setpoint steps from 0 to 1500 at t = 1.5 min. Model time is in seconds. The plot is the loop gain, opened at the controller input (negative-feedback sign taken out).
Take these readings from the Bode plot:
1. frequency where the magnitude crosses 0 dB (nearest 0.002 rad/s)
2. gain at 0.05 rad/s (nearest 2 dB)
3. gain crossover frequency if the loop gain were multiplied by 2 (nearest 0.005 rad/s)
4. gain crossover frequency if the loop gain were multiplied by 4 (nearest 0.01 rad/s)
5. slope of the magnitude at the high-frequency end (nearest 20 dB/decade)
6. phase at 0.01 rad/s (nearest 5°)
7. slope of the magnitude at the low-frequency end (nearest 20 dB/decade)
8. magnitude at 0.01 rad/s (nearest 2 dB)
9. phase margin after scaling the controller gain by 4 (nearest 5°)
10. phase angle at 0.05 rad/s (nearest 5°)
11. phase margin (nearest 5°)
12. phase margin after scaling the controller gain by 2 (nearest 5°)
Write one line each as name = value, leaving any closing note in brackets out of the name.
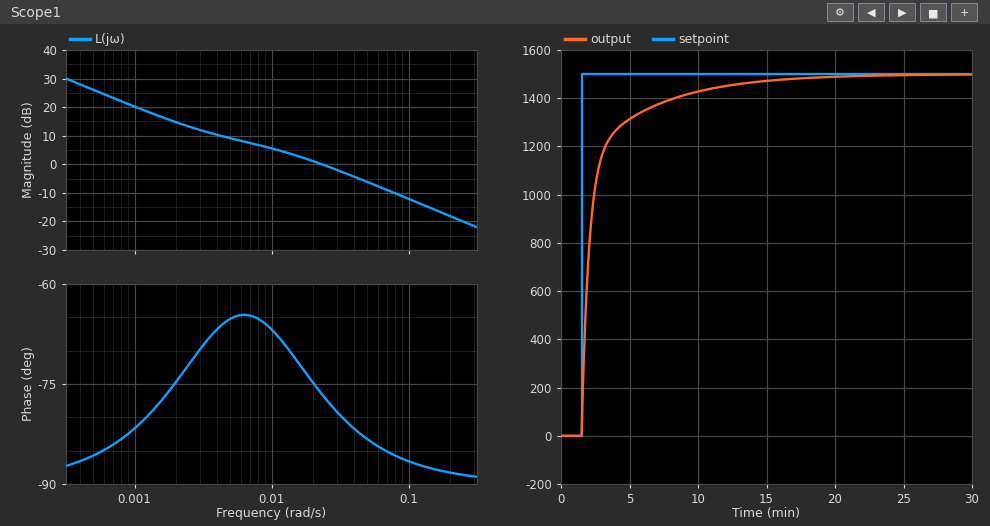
frequency where the magnitude crosses 0 dB = 0.024 rad/s
gain at 0.05 rad/s = -6 dB
gain crossover frequency if the loop gain were multiplied by 2 = 0.050 rad/s
gain crossover frequency if the loop gain were multiplied by 4 = 0.10 rad/s
slope of the magnitude at the high-frequency end = -20 dB/decade
phase at 0.01 rad/s = -65°
slope of the magnitude at the low-frequency end = -20 dB/decade
magnitude at 0.01 rad/s = 6 dB
phase margin after scaling the controller gain by 4 = 95°
phase angle at 0.05 rad/s = -85°
phase margin = 105°
phase margin after scaling the controller gain by 2 = 95°
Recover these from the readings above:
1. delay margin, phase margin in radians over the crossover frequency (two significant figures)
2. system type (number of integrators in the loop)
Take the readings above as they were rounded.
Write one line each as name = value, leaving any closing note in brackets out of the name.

delay margin, phase margin in radians over the crossover frequency = 76 s
system type = 1
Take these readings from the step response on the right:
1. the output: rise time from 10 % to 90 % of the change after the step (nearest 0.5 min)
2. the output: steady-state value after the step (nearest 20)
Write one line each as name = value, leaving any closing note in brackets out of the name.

the output: rise time from 10 % to 90 % of the change after the step = 4.5 min
the output: steady-state value after the step = 1500
